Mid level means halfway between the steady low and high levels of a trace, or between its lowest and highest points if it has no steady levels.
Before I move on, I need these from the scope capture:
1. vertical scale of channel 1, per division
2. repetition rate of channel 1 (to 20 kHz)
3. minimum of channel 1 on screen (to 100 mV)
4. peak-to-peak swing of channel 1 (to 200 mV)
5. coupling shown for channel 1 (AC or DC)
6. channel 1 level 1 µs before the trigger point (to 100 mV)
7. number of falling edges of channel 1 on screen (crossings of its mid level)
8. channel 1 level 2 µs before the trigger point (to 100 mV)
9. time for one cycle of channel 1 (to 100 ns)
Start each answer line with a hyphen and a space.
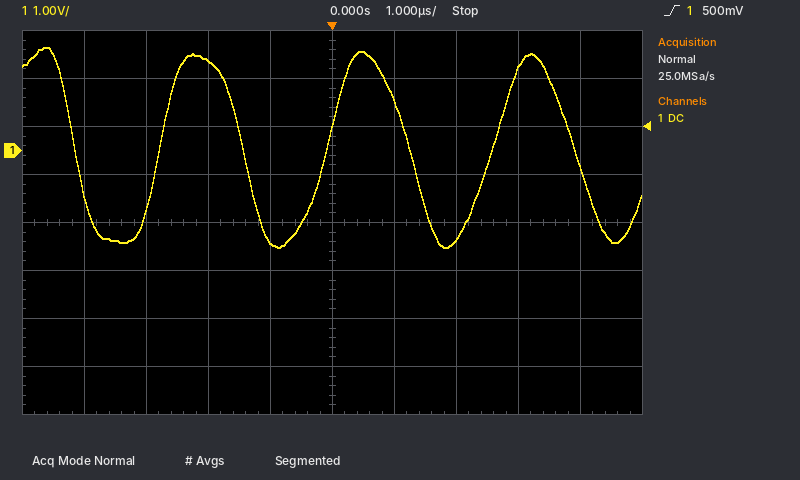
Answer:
- 1 V
- 380 kHz
- -2.0 V
- 4.2 V
- DC
- -1.9 V
- 4
- 1.9 V
- 2.7 µs
